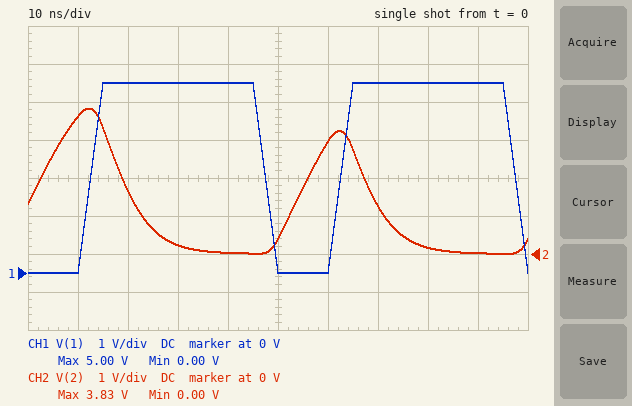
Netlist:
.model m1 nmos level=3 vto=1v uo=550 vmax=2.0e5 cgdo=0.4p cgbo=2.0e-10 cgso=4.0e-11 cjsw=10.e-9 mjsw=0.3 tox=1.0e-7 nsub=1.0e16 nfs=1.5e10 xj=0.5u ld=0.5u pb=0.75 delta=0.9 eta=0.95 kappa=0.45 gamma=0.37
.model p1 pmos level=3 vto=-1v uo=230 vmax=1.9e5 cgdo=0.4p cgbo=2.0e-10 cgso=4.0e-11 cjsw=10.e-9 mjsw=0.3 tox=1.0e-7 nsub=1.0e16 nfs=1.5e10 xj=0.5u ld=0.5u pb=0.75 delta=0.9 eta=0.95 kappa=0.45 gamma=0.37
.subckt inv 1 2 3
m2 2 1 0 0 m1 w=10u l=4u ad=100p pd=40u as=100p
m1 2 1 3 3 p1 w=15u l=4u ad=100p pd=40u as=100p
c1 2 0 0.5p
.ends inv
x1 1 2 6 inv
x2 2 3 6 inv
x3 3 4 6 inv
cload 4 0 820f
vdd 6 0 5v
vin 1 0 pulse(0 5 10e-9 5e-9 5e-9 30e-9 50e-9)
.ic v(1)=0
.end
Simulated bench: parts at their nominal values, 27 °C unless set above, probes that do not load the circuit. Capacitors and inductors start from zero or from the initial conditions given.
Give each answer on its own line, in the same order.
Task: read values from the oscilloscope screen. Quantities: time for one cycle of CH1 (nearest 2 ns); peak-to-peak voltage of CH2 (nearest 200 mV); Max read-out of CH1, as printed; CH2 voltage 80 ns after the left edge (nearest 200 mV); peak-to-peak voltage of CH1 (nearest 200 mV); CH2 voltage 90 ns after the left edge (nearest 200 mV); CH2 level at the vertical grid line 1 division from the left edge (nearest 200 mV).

50 ns
3.8 V
5.00 V
200 mV
5.0 V
0 V
3.6 V
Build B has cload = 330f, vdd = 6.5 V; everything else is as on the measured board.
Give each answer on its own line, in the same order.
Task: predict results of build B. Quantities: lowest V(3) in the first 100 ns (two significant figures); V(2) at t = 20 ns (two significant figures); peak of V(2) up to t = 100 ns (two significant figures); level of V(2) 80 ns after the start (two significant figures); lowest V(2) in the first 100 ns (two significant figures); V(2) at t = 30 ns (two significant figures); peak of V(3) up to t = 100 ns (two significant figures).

230 mV
3.3 V
5.7 V
620 mV
96 mV
680 mV
6.4 V
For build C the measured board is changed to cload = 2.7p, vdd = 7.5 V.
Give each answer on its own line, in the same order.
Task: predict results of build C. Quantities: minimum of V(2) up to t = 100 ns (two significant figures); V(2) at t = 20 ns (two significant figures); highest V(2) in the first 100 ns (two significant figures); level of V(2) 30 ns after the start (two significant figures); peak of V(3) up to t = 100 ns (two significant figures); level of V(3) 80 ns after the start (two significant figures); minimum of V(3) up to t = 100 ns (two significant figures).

380 mV
4.5 V
6.9 V
1.5 V
7.3 V
2.6 V
110 mV
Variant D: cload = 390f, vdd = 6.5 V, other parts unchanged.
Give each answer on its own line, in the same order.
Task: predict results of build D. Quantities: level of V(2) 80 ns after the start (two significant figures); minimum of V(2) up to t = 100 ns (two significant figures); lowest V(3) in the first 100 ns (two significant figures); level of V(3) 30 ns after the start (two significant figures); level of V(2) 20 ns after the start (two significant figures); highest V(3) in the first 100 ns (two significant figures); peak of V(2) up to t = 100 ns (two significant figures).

620 mV
96 mV
230 mV
2.8 V
3.3 V
6.4 V
5.7 V
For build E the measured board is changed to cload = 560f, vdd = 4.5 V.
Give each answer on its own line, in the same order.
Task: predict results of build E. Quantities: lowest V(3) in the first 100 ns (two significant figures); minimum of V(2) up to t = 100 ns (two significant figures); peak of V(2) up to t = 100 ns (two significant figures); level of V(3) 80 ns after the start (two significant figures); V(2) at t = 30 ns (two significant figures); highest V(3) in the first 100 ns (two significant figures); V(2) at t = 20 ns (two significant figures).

780 mV
-2.6 mV
3.2 V
4.3 V
160 mV
4.5 V
1.2 V
